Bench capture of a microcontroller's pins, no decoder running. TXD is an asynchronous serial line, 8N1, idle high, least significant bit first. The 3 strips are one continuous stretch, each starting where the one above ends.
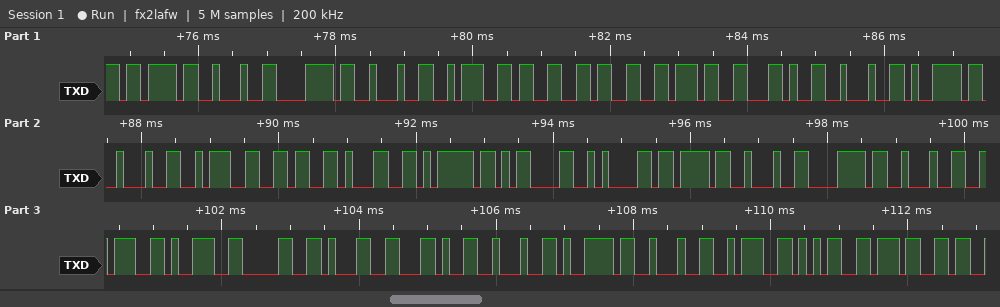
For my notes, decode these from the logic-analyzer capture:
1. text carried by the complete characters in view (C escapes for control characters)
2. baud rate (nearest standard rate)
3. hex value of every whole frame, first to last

"{\"x\":337,\"y\":61}\r\n{\"x\":901,\"y\":57"
9600 baud
7B 22 78 22 3A 33 33 37 2C 22 79 22 3A 36 31 7D 0D 0A 7B 22 78 22 3A 39 30 31 2C 22 79 22 3A 35 37
